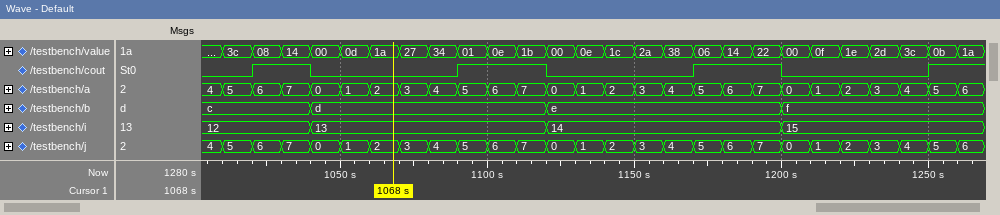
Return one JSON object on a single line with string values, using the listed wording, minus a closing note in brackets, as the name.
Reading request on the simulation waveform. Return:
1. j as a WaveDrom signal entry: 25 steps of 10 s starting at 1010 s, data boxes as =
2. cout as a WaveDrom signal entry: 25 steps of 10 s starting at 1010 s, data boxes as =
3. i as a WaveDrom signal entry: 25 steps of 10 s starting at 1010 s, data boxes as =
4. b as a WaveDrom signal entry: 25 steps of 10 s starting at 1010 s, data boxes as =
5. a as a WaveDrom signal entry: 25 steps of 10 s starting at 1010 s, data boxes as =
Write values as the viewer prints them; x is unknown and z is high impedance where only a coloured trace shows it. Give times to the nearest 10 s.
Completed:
{"j as a WaveDrom signal entry: 25 steps of 10 s starting at 1010 s, data boxes as =": "{name: 'j', wave: '=========================', data: '5 6 7 0 1 2 3 4 5 6 7 0 1 2 3 4 5 6 7 0 1 2 3 4 5'}", "cout as a WaveDrom signal entry: 25 steps of 10 s starting at 1010 s, data boxes as =": "{name: 'cout', wave: '01.0....1..0....1..0....1'}", "i as a WaveDrom signal entry: 25 steps of 10 s starting at 1010 s, data boxes as =": "{name: 'i', wave: '=..=.......=.......=.....', data: '12 13 14 15'}", "b as a WaveDrom signal entry: 25 steps of 10 s starting at 1010 s, data boxes as =": "{name: 'b', wave: '=..=.......=.......=.....', data: 'c d e f'}", "a as a WaveDrom signal entry: 25 steps of 10 s starting at 1010 s, data boxes as =": "{name: 'a', wave: '=========================', data: '5 6 7 0 1 2 3 4 5 6 7 0 1 2 3 4 5 6 7 0 1 2 3 4 5'}"}
